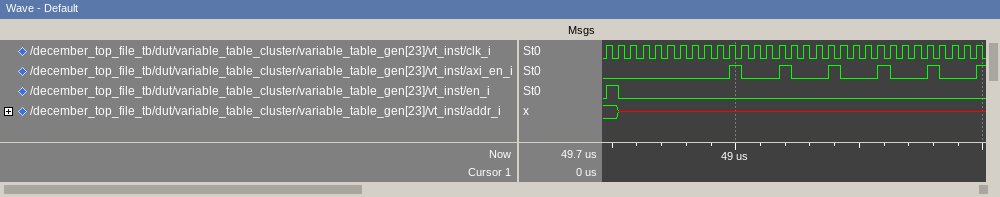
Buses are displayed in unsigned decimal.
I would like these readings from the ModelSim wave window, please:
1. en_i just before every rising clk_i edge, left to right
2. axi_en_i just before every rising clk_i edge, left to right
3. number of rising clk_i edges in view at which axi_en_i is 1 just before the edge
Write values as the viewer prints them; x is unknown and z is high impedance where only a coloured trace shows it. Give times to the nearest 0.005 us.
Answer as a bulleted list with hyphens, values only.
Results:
- 0 1 0 0 0 0 0 0 0 0 0 0 0 0 0 0 0 0 0 0 0 0 0 0 0 0 0 0 0 0 0
- 0 0 0 0 0 0 0 0 0 0 0 1 0 0 0 1 0 0 0 1 0 0 0 1 0 0 0 1 0 0 0
- 5
